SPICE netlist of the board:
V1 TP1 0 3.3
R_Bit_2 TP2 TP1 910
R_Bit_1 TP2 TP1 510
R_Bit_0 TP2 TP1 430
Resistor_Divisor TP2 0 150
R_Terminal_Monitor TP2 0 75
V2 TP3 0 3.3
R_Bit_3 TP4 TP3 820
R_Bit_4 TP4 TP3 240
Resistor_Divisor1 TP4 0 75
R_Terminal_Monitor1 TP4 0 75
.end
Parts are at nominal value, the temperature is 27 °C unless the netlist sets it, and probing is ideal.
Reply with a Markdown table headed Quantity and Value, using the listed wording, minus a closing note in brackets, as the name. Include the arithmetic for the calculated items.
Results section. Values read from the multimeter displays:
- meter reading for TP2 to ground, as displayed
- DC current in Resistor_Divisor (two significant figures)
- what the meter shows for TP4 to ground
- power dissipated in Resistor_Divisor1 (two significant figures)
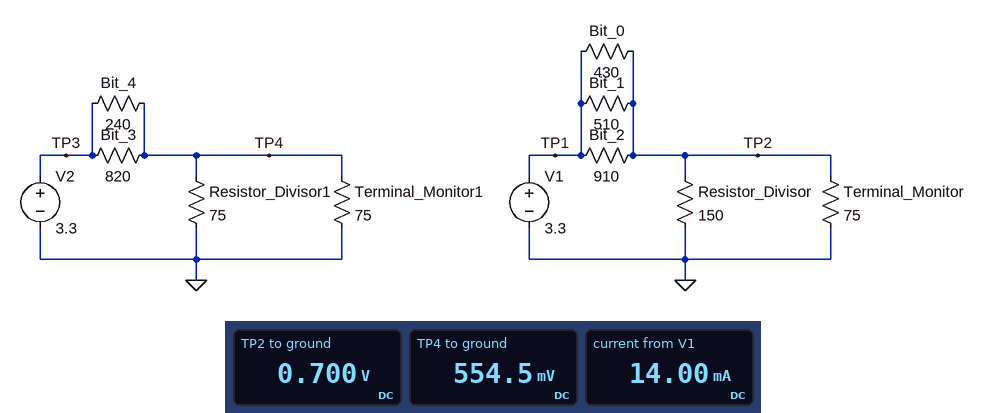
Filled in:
| Quantity | Value |
|---|---|
| meter reading for TP2 to ground, as displayed | 0.700 V |
| DC current in Resistor_Divisor | (700 mV) / 150 Ω = 4.7 mA |
| what the meter shows for TP4 to ground | 554.5 mV |
| power dissipated in Resistor_Divisor1 | (554.5 mV)^2 / 75 Ω = 4.1 mW |
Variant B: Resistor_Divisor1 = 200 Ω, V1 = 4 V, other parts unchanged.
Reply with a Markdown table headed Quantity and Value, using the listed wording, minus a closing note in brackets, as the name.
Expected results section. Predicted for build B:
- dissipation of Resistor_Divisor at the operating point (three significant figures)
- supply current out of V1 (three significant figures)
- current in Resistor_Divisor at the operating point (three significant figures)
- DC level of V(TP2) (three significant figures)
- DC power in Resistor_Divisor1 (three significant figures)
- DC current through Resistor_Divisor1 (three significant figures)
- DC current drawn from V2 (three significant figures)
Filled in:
| Quantity | Value |
|---|---|
| dissipation of Resistor_Divisor at the operating point | 4.80 mW |
| supply current out of V1 | 17.0 mA |
| current in Resistor_Divisor at the operating point | 5.66 mA |
| DC level of V(TP2) | 849 mV |
| DC power in Resistor_Divisor1 | 2.81 mW |
| DC current through Resistor_Divisor1 | 3.75 mA |
| DC current drawn from V2 | 13.7 mA |
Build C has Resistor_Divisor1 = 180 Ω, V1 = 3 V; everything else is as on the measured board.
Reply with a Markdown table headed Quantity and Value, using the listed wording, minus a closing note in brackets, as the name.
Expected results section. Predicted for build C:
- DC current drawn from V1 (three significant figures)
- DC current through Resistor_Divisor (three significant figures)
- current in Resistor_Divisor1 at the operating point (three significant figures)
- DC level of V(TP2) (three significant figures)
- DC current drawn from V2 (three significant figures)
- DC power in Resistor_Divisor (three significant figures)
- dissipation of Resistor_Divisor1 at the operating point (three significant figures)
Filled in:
| Quantity | Value |
|---|---|
| DC current drawn from V1 | 12.7 mA |
| DC current through Resistor_Divisor | 4.24 mA |
| current in Resistor_Divisor1 at the operating point | 4.07 mA |
| DC level of V(TP2) | 636 mV |
| DC current drawn from V2 | 13.8 mA |
| DC power in Resistor_Divisor | 2.70 mW |
| dissipation of Resistor_Divisor1 at the operating point | 2.98 mW |
